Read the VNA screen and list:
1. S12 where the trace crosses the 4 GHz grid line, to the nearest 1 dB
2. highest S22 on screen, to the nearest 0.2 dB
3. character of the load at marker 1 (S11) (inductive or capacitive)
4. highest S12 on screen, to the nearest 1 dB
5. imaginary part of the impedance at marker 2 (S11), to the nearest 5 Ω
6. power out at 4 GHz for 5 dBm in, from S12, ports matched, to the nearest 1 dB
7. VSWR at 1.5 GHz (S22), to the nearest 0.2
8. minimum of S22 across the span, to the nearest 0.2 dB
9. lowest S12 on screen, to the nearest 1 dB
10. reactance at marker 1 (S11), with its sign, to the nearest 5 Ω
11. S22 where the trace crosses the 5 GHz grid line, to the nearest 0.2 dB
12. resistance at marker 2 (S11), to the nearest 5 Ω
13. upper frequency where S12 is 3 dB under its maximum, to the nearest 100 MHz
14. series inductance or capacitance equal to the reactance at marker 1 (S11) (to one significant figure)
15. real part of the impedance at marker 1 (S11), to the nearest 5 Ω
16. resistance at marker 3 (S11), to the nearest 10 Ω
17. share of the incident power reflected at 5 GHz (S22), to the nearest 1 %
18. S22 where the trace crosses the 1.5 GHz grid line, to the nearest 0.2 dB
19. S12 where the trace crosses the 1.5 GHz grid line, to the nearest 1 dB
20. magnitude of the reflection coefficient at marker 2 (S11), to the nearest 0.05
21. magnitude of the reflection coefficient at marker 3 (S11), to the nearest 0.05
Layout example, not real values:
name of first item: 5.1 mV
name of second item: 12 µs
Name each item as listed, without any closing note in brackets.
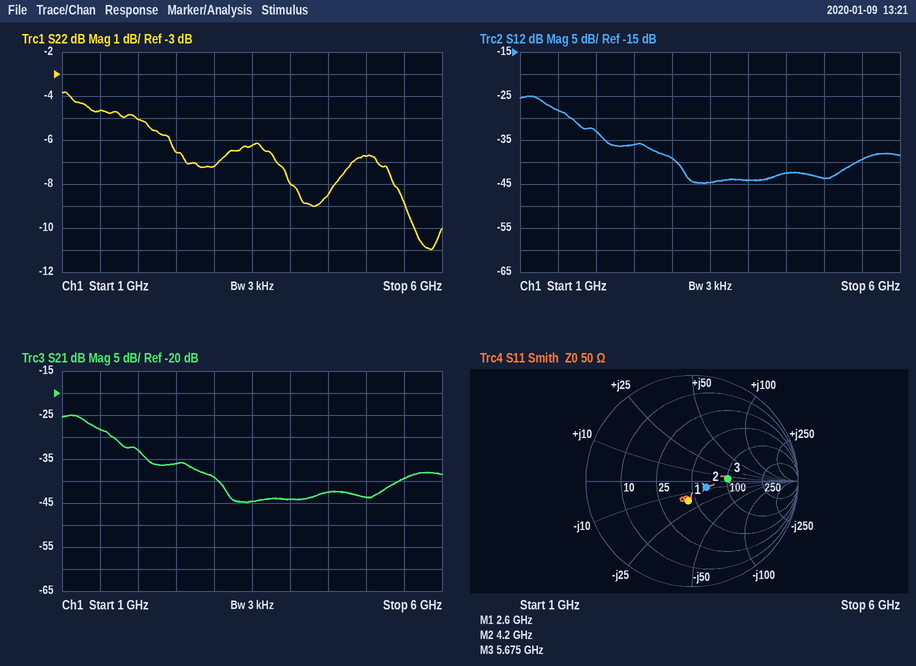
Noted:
S12 where the trace crosses the 4 GHz grid line, to the nearest 1 dB: -44 dB
highest S22 on screen, to the nearest 0.2 dB: -3.8 dB
character of the load at marker 1 (S11): capacitive
highest S12 on screen, to the nearest 1 dB: -25 dB
imaginary part of the impedance at marker 2 (S11), to the nearest 5 Ω: -10 Ω
power out at 4 GHz for 5 dBm in, from S12, ports matched, to the nearest 1 dB: -39 dBm
VSWR at 1.5 GHz (S22), to the nearest 0.2: 3.8
minimum of S22 across the span, to the nearest 0.2 dB: -11.0 dB
lowest S12 on screen, to the nearest 1 dB: -45 dB
reactance at marker 1 (S11), with its sign, to the nearest 5 Ω: -15 Ω
S22 where the trace crosses the 5 GHz grid line, to the nearest 0.2 dB: -6.8 dB
resistance at marker 2 (S11), to the nearest 5 Ω: 65 Ω
upper frequency where S12 is 3 dB under its maximum, to the nearest 100 MHz: 1.5 GHz
series inductance or capacitance equal to the reactance at marker 1 (S11): 4 pF
real part of the impedance at marker 1 (S11), to the nearest 5 Ω: 45 Ω
resistance at marker 3 (S11), to the nearest 10 Ω: 100 Ω
share of the incident power reflected at 5 GHz (S22), to the nearest 1 %: 21 %
S22 where the trace crosses the 1.5 GHz grid line, to the nearest 0.2 dB: -4.6 dB
S12 where the trace crosses the 1.5 GHz grid line, to the nearest 1 dB: -28 dB
magnitude of the reflection coefficient at marker 2 (S11), to the nearest 0.05: 0.15
magnitude of the reflection coefficient at marker 3 (S11), to the nearest 0.05: 0.35
